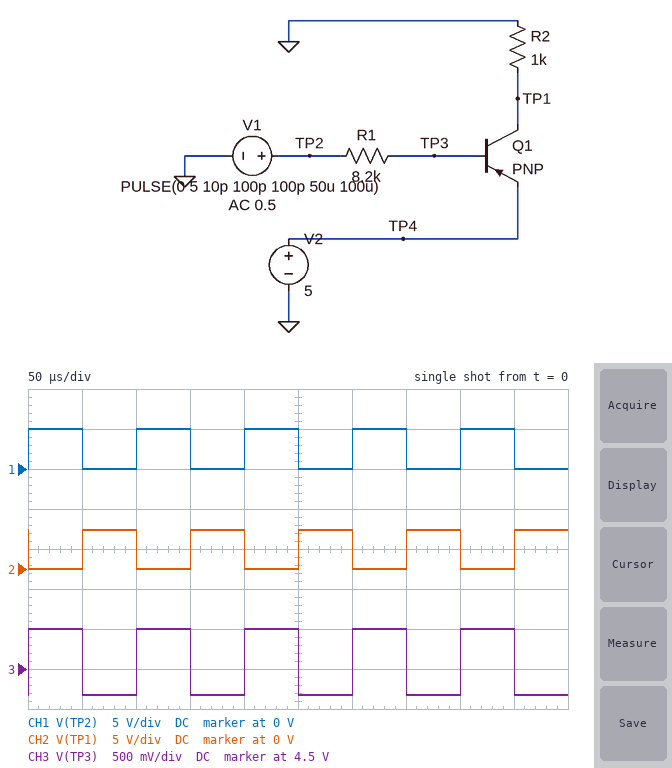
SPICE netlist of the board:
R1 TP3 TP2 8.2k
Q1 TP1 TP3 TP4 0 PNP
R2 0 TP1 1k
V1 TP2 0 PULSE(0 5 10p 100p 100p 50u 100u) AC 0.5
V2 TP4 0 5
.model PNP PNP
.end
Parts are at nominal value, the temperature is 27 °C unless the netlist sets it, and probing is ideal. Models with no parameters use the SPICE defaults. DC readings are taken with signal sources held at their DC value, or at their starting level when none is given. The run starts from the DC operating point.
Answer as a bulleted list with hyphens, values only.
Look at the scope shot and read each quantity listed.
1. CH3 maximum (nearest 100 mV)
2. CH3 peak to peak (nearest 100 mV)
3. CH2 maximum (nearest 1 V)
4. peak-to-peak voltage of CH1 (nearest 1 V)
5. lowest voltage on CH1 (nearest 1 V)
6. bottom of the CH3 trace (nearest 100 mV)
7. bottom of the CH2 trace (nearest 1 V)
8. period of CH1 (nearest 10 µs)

- 5.0 V
- 800 mV
- 5 V
- 5 V
- 0 V
- 4.2 V
- 0 V
- 100 µs
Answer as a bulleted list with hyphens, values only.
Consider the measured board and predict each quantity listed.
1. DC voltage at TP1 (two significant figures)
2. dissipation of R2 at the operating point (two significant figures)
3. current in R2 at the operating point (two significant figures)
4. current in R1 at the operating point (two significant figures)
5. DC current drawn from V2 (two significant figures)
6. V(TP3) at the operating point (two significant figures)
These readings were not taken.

- 4.9 V
- 24 mW
- 4.9 mA
- 510 µA
- 5.4 mA
- 4.2 V
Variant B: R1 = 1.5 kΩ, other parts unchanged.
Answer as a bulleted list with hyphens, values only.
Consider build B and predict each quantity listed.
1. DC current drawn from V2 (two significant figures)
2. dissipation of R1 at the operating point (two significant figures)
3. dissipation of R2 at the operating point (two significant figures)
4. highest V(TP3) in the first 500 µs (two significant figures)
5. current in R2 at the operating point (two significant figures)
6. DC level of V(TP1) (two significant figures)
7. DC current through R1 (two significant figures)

- 7.7 mA
- 12 mW
- 25 mW
- 5.0 V
- 5.0 mA
- 5.0 V
- 2.8 mA
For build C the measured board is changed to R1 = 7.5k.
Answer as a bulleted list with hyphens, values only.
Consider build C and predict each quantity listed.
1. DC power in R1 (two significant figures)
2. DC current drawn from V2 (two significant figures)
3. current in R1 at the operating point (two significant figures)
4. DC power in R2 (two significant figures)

- 2.3 mW
- 5.5 mA
- 560 µA
- 24 mW
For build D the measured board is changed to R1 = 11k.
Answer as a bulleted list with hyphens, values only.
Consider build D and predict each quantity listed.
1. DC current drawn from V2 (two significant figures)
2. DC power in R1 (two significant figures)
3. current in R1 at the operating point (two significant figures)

- 5.3 mA
- 1.6 mW
- 380 µA
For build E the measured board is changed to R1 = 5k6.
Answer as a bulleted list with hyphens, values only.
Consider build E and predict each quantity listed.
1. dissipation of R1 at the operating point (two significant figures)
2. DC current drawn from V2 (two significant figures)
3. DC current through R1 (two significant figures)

- 3.1 mW
- 5.7 mA
- 750 µA
